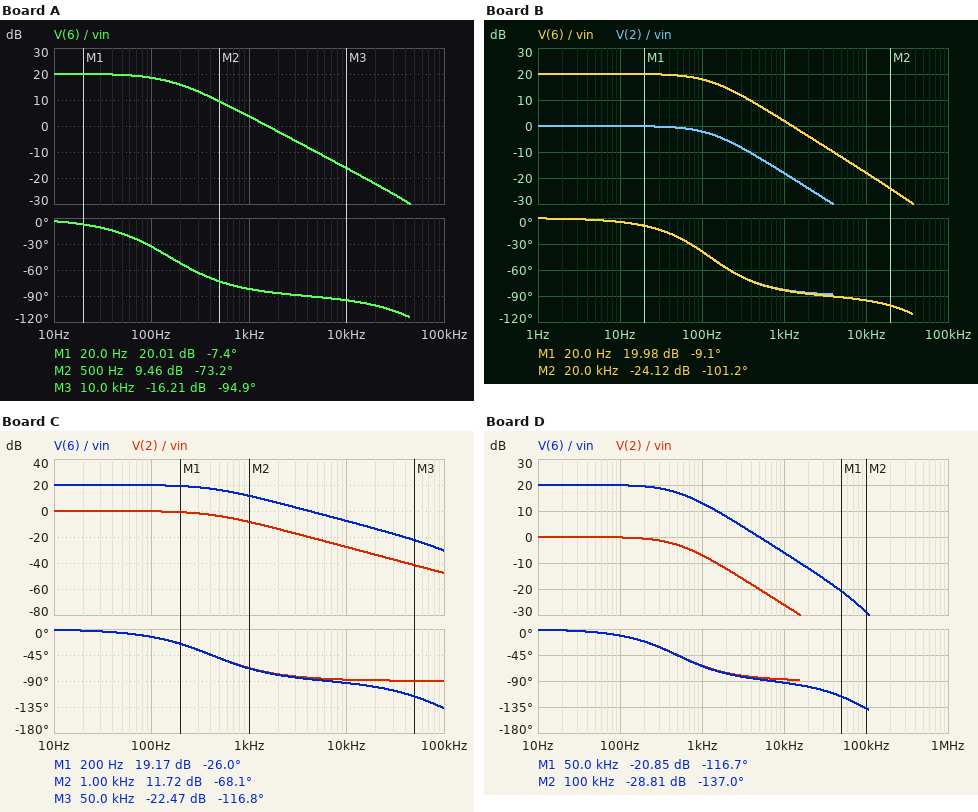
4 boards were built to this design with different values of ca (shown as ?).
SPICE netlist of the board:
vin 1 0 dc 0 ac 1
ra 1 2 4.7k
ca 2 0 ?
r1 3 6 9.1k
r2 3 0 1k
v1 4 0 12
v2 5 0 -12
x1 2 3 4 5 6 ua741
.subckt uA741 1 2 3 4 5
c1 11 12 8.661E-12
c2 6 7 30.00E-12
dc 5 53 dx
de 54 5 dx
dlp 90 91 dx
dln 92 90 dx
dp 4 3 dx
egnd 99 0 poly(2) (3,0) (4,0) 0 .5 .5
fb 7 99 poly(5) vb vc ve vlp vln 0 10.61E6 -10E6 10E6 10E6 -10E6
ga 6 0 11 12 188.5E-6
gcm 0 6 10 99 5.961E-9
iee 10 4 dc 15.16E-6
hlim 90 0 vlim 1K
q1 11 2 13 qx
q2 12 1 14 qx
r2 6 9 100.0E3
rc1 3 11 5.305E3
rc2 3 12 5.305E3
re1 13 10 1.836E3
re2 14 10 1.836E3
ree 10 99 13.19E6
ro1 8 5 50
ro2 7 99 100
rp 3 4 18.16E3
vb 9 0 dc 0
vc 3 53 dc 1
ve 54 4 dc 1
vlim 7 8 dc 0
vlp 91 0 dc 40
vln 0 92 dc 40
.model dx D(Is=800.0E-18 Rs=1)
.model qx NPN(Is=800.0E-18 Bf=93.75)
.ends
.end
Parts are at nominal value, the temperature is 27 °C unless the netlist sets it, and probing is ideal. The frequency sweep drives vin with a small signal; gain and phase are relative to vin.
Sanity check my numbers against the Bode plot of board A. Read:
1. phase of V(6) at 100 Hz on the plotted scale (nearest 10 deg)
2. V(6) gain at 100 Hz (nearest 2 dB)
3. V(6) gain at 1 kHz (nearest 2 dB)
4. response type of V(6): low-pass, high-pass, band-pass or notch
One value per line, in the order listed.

-30 deg
18 dB
4 dB
low-pass
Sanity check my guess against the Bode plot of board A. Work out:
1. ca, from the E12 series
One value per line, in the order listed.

220 nF
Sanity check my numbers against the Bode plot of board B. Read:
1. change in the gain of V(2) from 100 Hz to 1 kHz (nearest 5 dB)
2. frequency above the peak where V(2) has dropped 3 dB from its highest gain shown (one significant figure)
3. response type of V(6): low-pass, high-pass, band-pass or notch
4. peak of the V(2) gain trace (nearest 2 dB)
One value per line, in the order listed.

-15 dB
100 Hz
low-pass
0 dB
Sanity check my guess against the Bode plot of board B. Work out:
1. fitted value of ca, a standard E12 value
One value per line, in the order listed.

270 nF
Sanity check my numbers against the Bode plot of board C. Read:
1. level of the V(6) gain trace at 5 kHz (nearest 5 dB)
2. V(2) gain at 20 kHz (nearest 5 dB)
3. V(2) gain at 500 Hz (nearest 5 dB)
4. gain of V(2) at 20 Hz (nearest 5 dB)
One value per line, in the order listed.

0 dB
-35 dB
-5 dB
0 dB
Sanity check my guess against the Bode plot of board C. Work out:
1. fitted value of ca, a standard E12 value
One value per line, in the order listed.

82 nF
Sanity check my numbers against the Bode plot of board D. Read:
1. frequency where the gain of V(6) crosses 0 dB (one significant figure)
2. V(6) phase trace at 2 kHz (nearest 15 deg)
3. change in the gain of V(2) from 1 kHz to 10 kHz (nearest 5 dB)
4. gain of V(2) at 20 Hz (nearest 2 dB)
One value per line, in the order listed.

5 kHz
-75 deg
-20 dB
0 dB
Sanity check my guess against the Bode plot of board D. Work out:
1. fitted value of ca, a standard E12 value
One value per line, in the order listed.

68 nF
